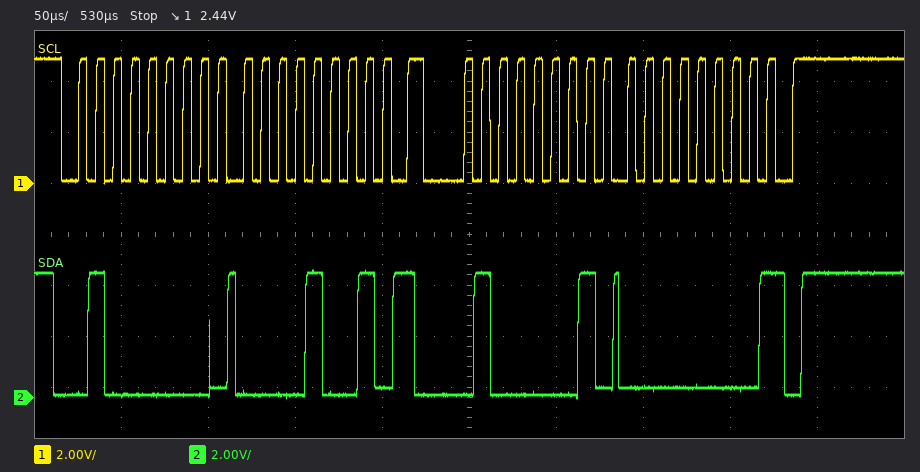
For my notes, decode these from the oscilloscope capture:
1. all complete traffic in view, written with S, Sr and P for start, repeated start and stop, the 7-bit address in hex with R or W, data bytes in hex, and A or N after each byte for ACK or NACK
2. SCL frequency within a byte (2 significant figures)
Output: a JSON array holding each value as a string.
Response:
["S 20W A 09 A Sr 20R A 00 N P", "100 kHz"]
